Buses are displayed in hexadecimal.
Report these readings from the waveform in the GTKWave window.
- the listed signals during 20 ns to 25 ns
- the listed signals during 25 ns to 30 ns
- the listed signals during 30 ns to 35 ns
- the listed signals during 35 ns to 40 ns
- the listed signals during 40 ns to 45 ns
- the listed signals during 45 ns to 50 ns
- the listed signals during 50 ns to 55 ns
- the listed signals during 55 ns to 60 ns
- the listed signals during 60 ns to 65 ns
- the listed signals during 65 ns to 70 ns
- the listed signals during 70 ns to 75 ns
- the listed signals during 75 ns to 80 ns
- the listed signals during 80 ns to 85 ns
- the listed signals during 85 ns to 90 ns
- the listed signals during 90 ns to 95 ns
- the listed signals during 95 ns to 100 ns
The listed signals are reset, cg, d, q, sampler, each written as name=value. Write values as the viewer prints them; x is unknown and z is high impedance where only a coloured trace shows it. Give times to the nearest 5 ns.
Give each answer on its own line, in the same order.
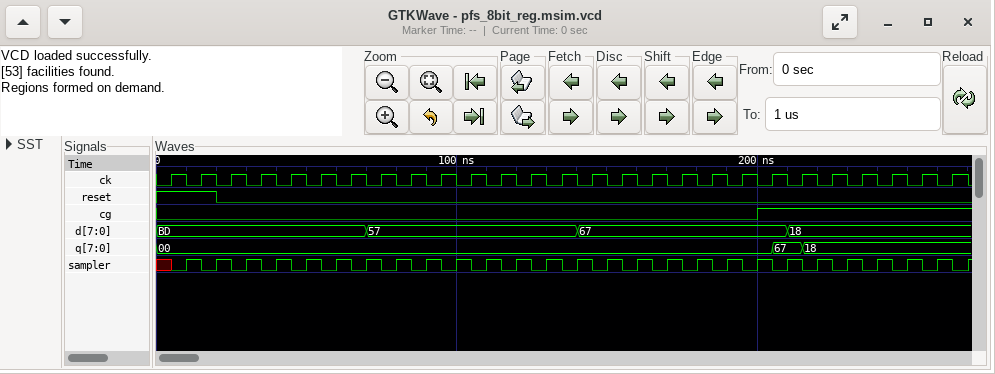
reset=0, cg=0, d=BD, q=00, sampler=1
reset=0, cg=0, d=BD, q=00, sampler=0
reset=0, cg=0, d=BD, q=00, sampler=1
reset=0, cg=0, d=BD, q=00, sampler=0
reset=0, cg=0, d=BD, q=00, sampler=1
reset=0, cg=0, d=BD, q=00, sampler=0
reset=0, cg=0, d=BD, q=00, sampler=1
reset=0, cg=0, d=BD, q=00, sampler=0
reset=0, cg=0, d=BD, q=00, sampler=1
reset=0, cg=0, d=BD, q=00, sampler=0
reset=0, cg=0, d=57, q=00, sampler=1
reset=0, cg=0, d=57, q=00, sampler=0
reset=0, cg=0, d=57, q=00, sampler=1
reset=0, cg=0, d=57, q=00, sampler=0
reset=0, cg=0, d=57, q=00, sampler=1
reset=0, cg=0, d=57, q=00, sampler=0
